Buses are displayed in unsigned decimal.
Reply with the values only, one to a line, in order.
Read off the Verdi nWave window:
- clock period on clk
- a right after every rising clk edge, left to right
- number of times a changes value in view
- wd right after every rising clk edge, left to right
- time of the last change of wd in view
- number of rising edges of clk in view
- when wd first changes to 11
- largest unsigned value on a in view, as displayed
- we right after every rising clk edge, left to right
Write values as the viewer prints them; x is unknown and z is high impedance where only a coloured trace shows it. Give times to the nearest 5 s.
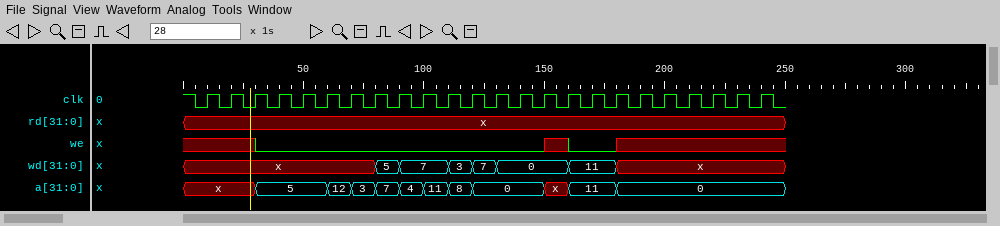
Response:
10 s
x, x, 5, 5, 5, 12, 3, 7, 4, 11, 8, 0, 0, 0, x, 11, 11, 0, 0, 0, 0, 0, 0, 0
11
x, x, x, x, x, x, x, 5, 7, 7, 3, 7, 0, 0, 0, 11, 11, x, x, x, x, x, x, x
180 s
24
160 s
12
x x 0 0 0 0 0 0 0 0 0 0 0 0 x 0 0 x x x x x x x
